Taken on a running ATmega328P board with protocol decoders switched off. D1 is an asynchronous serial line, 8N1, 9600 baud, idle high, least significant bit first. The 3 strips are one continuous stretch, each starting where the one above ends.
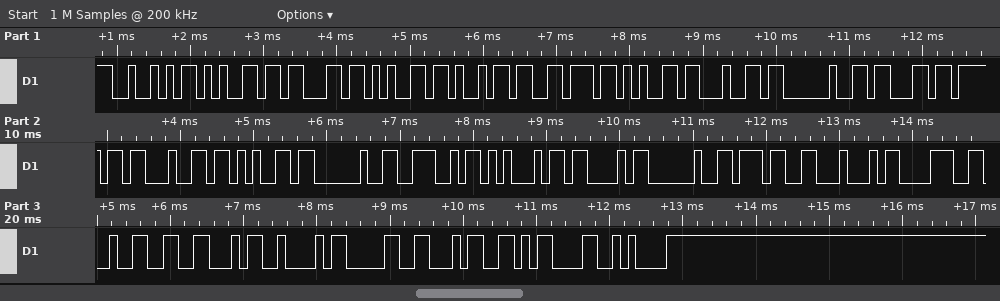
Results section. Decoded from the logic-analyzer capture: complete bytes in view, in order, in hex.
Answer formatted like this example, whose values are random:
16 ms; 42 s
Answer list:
0x52 0x65 0x63 0x65 0x69 0x76 0x65 0x64 0x20 0x63 0x6F 0x64 0x65 0x20 0x4E 0x45 0x43 0x20 0x37 0x44 0x38 0x32 0x46 0x42 0x30 0x34 0x0D 0x0A
